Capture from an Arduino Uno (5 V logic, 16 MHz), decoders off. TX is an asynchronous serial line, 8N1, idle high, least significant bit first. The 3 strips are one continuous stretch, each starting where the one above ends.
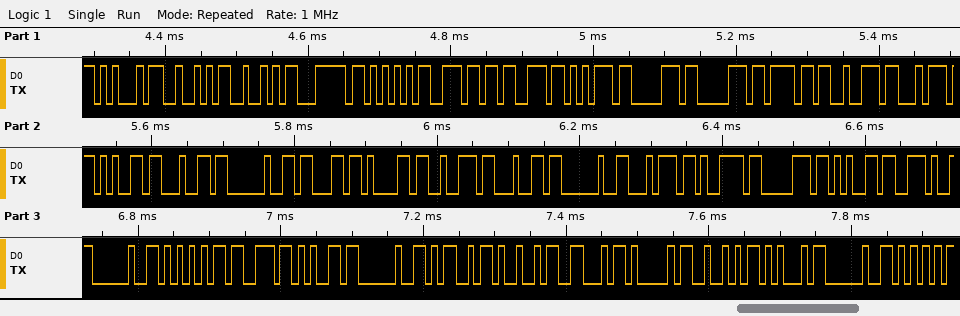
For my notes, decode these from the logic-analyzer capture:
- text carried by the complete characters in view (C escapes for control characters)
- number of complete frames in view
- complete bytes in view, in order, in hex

"ERR|Unsupported card type. Use MIFARE U"
39
0x45 0x52 0x52 0x7C 0x55 0x6E 0x73 0x75 0x70 0x70 0x6F 0x72 0x74 0x65 0x64 0x20 0x63 0x61 0x72 0x64 0x20 0x74 0x79 0x70 0x65 0x2E 0x20 0x55 0x73 0x65 0x20 0x4D 0x49 0x46 0x41 0x52 0x45 0x20 0x55
